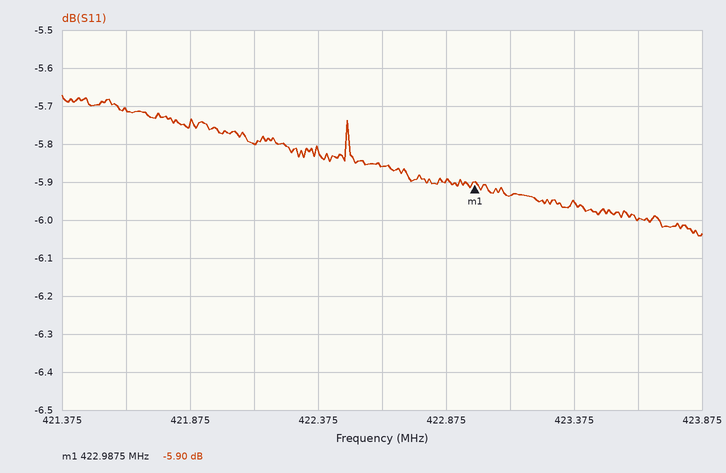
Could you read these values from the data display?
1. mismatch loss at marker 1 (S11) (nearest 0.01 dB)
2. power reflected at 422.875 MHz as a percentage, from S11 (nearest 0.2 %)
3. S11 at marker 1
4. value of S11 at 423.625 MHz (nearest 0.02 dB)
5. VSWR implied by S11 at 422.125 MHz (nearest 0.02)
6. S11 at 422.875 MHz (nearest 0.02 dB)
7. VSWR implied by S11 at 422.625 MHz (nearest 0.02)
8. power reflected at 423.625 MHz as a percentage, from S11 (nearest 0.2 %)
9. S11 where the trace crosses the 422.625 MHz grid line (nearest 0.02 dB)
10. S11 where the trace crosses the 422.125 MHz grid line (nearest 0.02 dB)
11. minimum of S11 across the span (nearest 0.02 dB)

1.29 dB
25.8 %
-5.90 dB
-6.00 dB
3.10
-5.90 dB
3.08
25.2 %
-5.86 dB
-5.80 dB
-6.04 dB
